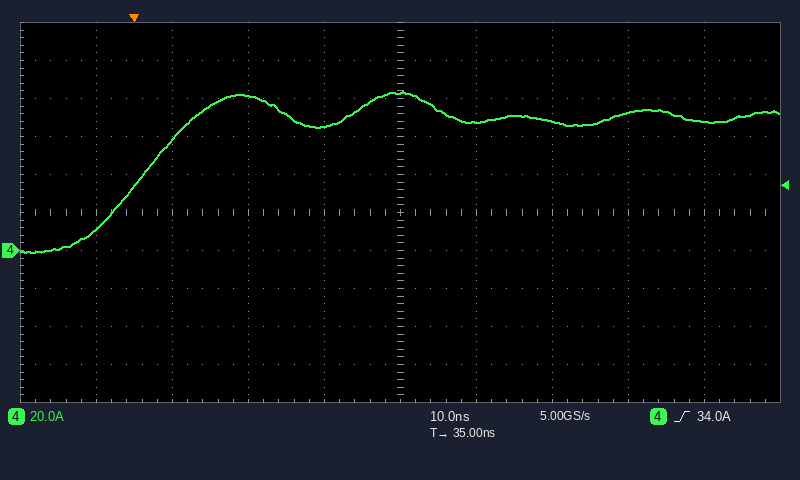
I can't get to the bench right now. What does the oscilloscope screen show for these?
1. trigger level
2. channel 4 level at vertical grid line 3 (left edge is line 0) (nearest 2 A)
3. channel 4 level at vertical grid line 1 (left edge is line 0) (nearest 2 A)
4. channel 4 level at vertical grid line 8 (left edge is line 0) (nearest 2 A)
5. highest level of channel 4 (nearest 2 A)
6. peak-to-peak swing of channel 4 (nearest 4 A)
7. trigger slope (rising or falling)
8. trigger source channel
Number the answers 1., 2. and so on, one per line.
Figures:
1. 34.0 A
2. 82 A
3. 12 A
4. 72 A
5. 84 A
6. 84 A
7. rising
8. channel 4
